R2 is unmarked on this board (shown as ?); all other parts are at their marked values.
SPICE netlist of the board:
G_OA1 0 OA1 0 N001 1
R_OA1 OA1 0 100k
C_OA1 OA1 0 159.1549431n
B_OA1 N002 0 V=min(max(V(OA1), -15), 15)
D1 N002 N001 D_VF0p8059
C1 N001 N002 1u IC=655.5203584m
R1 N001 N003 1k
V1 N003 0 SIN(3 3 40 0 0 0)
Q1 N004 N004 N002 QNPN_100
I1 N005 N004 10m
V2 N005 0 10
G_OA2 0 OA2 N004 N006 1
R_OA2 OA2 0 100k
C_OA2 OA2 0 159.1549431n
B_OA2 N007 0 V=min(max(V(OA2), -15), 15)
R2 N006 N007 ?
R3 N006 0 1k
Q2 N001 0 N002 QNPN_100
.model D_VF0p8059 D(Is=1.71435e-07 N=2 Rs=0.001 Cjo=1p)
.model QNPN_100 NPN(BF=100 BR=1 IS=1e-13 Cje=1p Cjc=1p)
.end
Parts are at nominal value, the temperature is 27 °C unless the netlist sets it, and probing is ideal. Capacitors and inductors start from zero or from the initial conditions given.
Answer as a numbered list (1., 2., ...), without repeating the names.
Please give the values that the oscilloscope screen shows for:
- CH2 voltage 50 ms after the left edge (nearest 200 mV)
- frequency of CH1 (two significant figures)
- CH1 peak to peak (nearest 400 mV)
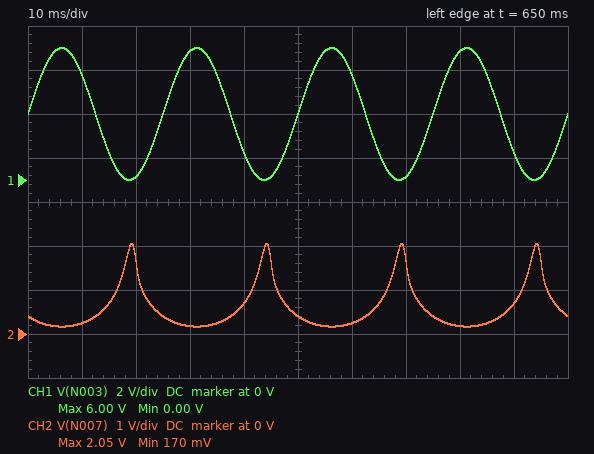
1. 400 mV
2. 40 Hz
3. 6.0 V
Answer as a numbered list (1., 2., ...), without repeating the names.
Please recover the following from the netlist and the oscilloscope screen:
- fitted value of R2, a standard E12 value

1. 12 kΩ
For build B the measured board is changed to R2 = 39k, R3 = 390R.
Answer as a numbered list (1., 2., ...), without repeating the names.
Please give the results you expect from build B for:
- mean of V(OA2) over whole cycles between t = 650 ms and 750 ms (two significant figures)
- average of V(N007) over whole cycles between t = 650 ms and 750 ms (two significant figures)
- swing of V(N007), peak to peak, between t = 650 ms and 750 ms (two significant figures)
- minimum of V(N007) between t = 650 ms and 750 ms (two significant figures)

1. 5.7 V
2. 4.7 V
3. 14 V
4. 1.3 V
